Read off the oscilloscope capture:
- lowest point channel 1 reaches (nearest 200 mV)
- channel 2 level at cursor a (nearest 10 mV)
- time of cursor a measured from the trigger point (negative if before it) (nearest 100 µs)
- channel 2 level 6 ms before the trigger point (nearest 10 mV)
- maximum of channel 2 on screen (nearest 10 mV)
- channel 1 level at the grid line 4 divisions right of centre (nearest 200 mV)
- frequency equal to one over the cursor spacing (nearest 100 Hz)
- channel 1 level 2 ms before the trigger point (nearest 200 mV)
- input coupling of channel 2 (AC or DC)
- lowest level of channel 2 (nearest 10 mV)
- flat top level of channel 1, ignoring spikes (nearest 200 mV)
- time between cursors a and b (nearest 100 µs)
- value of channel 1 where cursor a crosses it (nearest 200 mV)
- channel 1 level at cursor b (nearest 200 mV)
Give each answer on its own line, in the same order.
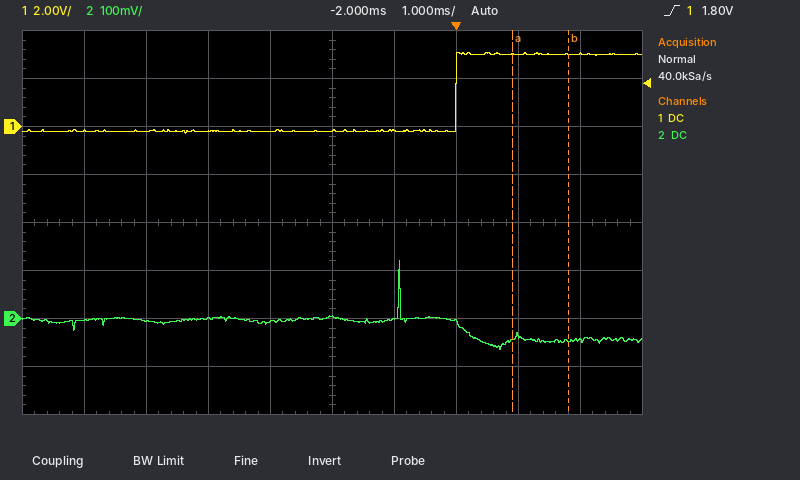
-200 mV
-40 mV
+900 µs
0 mV
120 mV
3.0 V
1.1 kHz
-200 mV
DC
-60 mV
3.0 V
900 µs
3.0 V
3.0 V
